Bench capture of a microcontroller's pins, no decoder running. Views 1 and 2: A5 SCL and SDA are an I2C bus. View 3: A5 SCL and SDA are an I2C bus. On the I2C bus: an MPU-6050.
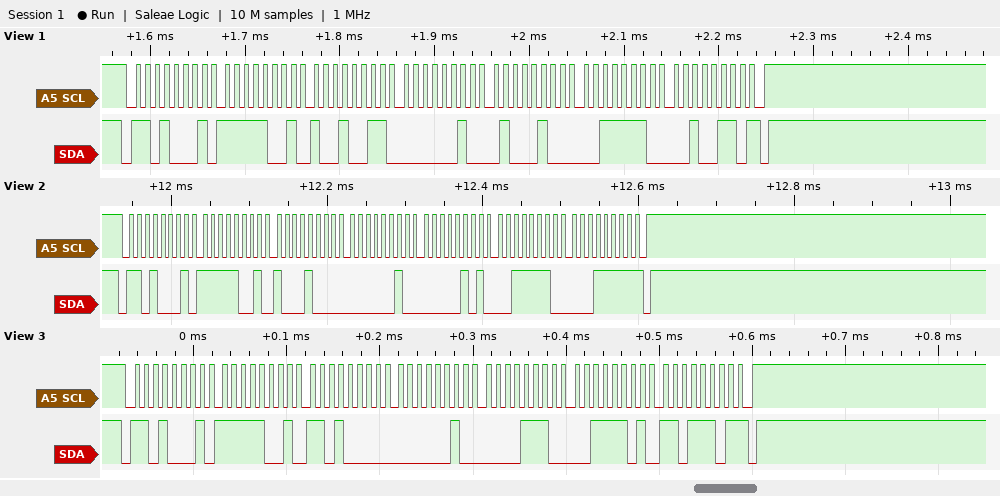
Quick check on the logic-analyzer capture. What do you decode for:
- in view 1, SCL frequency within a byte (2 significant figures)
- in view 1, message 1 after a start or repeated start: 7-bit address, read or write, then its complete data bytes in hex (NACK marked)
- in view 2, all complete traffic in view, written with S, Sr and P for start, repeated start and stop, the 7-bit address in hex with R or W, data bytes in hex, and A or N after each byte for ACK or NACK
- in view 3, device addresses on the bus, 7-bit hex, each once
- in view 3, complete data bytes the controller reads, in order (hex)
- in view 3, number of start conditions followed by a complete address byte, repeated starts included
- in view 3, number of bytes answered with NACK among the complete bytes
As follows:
100 kHz
0x68 read: F9 93 02 44 3E 26 NACK
S 68R A F9 A 88 A 02 A 05 A 3E A 1F N P
0x68
F9 D0 02 0E 3D DD
1
1
